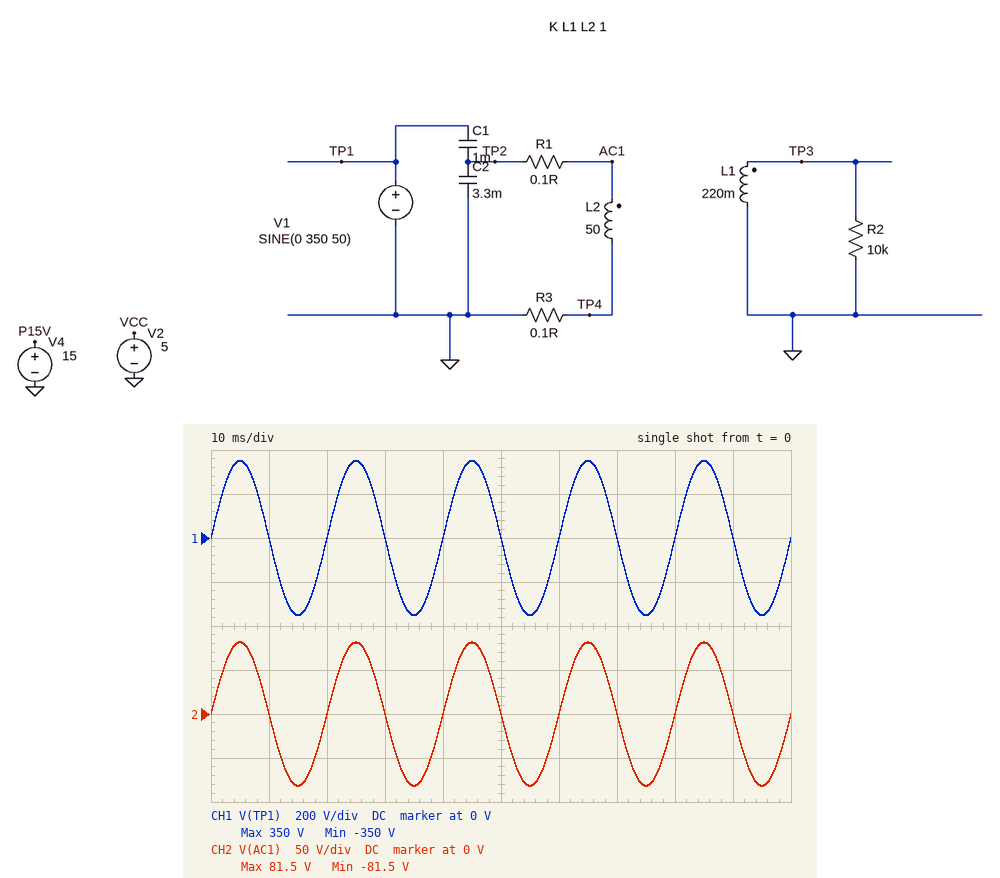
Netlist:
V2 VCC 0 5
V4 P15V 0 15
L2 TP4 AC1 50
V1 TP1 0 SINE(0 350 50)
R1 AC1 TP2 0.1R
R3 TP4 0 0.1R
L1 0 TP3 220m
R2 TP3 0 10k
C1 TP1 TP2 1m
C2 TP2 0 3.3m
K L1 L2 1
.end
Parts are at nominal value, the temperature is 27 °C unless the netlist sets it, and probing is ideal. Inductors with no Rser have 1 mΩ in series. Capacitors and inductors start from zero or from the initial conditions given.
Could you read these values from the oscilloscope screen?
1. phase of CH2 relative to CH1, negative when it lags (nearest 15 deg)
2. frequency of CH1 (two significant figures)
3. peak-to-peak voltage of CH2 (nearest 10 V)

0 deg
50 Hz
160 V
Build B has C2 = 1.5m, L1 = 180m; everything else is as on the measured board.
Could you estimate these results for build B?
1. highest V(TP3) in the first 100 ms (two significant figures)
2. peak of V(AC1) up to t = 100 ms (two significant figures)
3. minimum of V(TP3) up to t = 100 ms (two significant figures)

8.4 V
140 V
-8.4 V
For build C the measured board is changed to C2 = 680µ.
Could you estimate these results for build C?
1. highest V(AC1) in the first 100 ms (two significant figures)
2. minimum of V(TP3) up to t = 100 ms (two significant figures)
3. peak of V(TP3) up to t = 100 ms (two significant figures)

210 V
-14 V
14 V
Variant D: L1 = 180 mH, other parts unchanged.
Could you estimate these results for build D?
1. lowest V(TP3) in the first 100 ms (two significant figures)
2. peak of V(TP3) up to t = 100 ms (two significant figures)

-4.9 V
4.9 V
